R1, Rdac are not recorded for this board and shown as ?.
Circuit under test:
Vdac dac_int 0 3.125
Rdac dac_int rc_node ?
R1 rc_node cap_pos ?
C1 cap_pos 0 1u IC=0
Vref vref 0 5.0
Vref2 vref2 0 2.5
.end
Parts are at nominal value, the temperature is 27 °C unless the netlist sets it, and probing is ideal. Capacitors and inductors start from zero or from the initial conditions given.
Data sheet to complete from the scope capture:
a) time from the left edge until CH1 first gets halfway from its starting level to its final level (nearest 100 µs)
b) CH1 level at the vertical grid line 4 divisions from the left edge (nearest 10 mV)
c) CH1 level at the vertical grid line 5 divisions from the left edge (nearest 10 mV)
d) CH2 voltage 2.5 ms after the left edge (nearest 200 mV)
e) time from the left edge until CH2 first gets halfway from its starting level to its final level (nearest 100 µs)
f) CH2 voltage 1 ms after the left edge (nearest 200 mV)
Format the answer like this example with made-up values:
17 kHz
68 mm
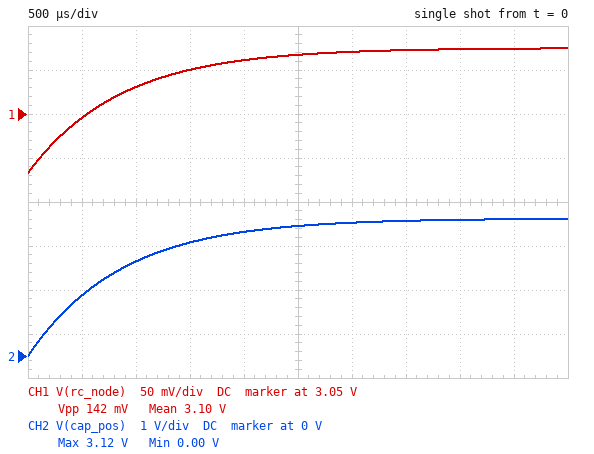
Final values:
600 µs
3.11 V
3.12 V
3.0 V
600 µs
2.2 V
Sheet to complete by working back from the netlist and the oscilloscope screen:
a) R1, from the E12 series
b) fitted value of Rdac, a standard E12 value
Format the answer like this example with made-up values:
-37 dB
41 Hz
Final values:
820 Ω
39 Ω
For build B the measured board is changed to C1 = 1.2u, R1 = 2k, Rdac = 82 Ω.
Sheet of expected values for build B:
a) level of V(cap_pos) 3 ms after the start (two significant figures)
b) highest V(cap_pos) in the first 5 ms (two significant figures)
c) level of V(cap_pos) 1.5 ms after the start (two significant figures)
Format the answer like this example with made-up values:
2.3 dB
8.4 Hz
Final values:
2.2 V
2.7 V
1.4 V
